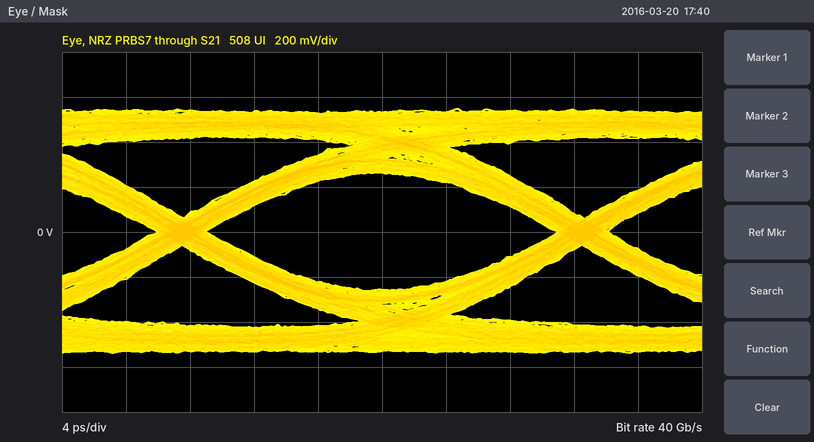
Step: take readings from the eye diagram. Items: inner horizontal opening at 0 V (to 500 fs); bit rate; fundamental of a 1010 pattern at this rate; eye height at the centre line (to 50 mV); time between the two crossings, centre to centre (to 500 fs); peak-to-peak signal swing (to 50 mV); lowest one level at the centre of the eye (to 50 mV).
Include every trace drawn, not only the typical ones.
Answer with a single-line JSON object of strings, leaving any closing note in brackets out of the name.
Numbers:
{"inner horizontal opening at 0 V": "22.0 ps", "bit rate": "40 Gb/s", "fundamental of a 1010 pattern at this rate": "20 GHz", "eye height at the centre line": "500 mV", "time between the two crossings, centre to centre": "25.0 ps", "peak-to-peak signal swing": "1.10 V", "lowest one level at the centre of the eye": "250 mV"}
